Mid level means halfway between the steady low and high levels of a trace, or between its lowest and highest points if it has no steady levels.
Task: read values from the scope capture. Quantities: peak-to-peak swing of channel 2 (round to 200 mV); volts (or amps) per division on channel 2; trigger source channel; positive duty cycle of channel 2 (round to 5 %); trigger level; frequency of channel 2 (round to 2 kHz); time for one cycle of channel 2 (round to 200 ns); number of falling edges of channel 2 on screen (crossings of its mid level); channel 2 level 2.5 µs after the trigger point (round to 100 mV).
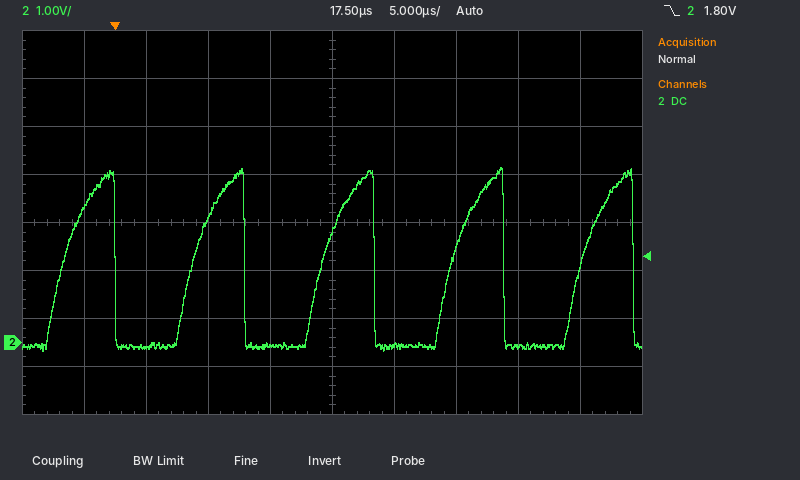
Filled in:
3.8 V
1 V
channel 2
40 %
1.80 V
96 kHz
10.4 µs
5
-100 mV
